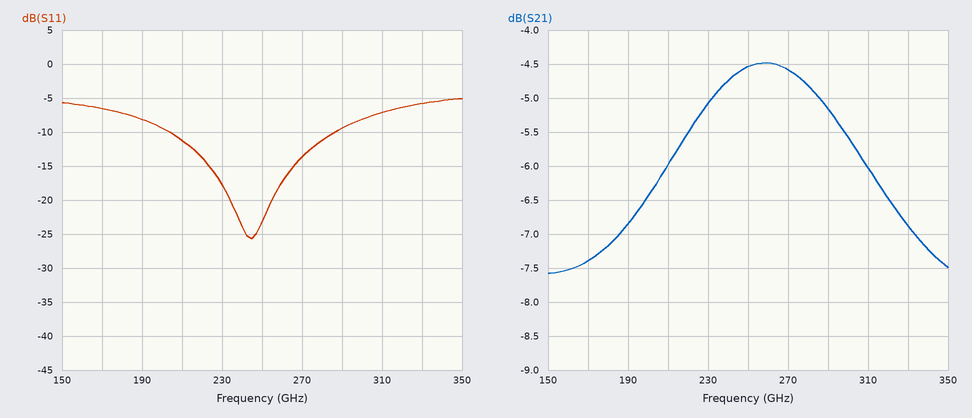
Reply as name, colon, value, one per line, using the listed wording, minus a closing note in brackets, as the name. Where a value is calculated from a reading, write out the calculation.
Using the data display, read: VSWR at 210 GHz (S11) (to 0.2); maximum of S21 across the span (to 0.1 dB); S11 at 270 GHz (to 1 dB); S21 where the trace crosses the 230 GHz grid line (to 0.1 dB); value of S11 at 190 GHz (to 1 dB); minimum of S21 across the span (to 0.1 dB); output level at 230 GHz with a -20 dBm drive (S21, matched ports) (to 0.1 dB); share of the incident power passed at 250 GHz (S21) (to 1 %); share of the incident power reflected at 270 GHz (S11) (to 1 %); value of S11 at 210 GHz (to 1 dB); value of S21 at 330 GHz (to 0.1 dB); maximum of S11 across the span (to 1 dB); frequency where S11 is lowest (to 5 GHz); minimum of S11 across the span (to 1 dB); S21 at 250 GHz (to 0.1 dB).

VSWR at 210 GHz (S11): |Γ| = 10^(-11/20) = 0.2818; VSWR = (1 + 0.2818)/(1 − 0.2818) ≈ 1.8
maximum of S21 across the span: -4.5 dB
S11 at 270 GHz: -14 dB
S21 where the trace crosses the 230 GHz grid line: -5.1 dB
value of S11 at 190 GHz: -8 dB
minimum of S21 across the span: -7.6 dB
output level at 230 GHz with a -20 dBm drive (S21, matched ports): -20 dBm + (-5.1 dB) = -25.1 dBm
share of the incident power passed at 250 GHz (S21): 10^(-4.5/10) ≈ 35 %
share of the incident power reflected at 270 GHz (S11): 10^(-14/10) ≈ 4 %
value of S11 at 210 GHz: -11 dB
value of S21 at 330 GHz: -6.9 dB
maximum of S11 across the span: -5 dB
frequency where S11 is lowest: 245 GHz
minimum of S11 across the span: -26 dB
S21 at 250 GHz: -4.5 dB
